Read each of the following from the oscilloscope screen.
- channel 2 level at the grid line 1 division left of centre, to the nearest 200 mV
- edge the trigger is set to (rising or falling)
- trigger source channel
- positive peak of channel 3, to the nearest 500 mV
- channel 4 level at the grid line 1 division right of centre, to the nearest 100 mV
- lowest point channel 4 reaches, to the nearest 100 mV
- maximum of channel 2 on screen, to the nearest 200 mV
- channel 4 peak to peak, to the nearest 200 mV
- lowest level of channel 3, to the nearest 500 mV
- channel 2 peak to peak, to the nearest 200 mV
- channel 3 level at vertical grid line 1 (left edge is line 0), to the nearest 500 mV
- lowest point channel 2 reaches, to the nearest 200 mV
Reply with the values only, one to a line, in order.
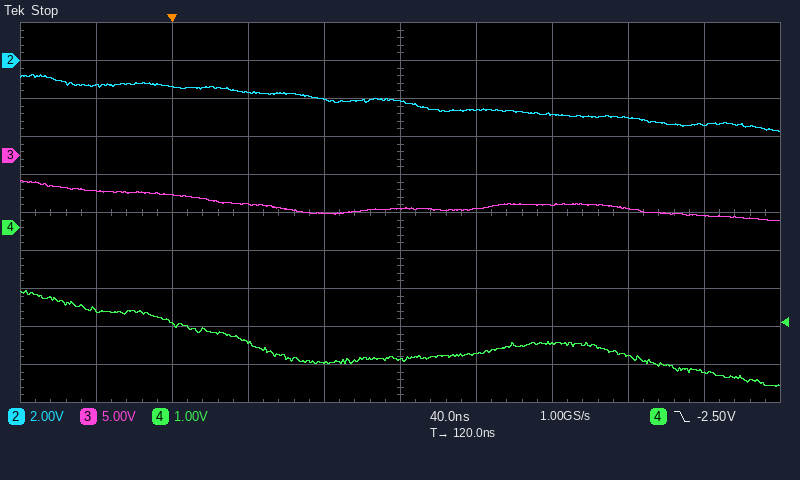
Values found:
-2.0 V
falling
channel 4
-3.5 V
-3.3 V
-4.2 V
-800 mV
2.6 V
-8.5 V
3.0 V
-4.5 V
-3.8 V
